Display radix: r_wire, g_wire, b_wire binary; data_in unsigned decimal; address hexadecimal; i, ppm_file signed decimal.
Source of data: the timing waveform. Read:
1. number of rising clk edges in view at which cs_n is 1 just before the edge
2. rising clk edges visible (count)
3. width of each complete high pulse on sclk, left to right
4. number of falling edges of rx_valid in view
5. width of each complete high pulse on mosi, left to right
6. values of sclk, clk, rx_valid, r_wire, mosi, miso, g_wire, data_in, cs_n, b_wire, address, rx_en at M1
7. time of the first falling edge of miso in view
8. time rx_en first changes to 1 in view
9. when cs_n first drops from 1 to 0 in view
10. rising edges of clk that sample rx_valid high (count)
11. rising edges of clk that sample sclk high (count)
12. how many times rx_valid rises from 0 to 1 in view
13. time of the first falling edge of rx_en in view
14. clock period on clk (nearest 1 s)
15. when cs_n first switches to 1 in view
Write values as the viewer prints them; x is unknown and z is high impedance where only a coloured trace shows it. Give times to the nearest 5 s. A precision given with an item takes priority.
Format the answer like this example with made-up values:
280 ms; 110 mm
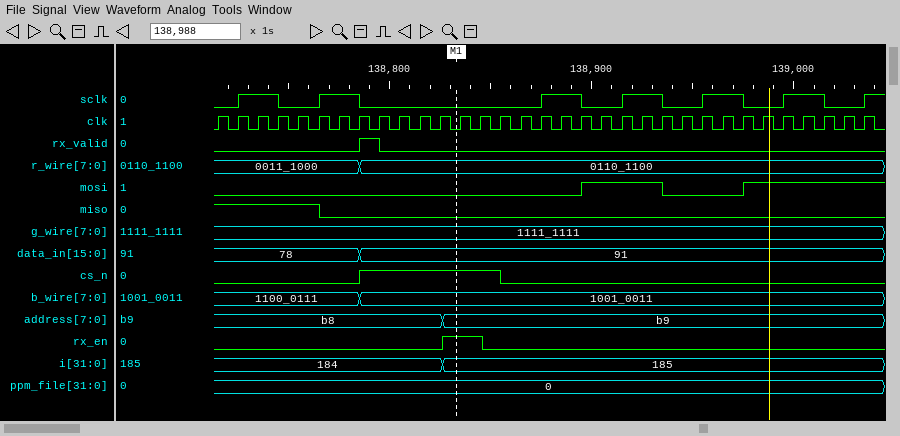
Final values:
7; 33; 20 s, 20 s, 20 s, 20 s, 20 s, 20 s; 1; 40 s; sclk=0, clk=0, rx_valid=0, r_wire=0110_1100, mosi=0, miso=0, g_wire=1111_1111, data_in=91, cs_n=1, b_wire=1001_0011, address=b9, rx_en=1; 138765 s; 138825 s; 138855 s; 1; 12; 1; 138845 s; 10 s; 138785 s
